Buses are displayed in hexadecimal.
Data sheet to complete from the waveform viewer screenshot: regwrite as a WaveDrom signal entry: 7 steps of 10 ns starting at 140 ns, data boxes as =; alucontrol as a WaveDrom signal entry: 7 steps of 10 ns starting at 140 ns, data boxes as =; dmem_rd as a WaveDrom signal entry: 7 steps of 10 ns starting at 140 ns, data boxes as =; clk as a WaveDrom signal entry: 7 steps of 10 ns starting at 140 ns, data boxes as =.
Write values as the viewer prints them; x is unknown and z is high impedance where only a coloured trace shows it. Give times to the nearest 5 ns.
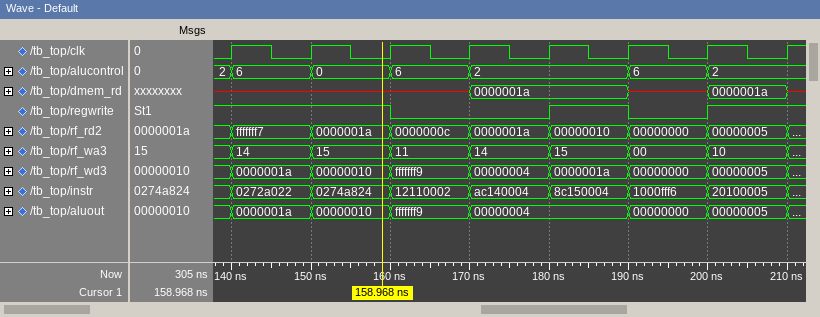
{name: 'regwrite', wave: '1.0.101'}
{name: 'alucontrol', wave: '====.==', data: '6 0 6 2 6 2'}
{name: 'dmem_rd', wave: 'x..=.x=', data: '0000001a 0000001a'}
{name: 'clk', wave: 'p......'}
